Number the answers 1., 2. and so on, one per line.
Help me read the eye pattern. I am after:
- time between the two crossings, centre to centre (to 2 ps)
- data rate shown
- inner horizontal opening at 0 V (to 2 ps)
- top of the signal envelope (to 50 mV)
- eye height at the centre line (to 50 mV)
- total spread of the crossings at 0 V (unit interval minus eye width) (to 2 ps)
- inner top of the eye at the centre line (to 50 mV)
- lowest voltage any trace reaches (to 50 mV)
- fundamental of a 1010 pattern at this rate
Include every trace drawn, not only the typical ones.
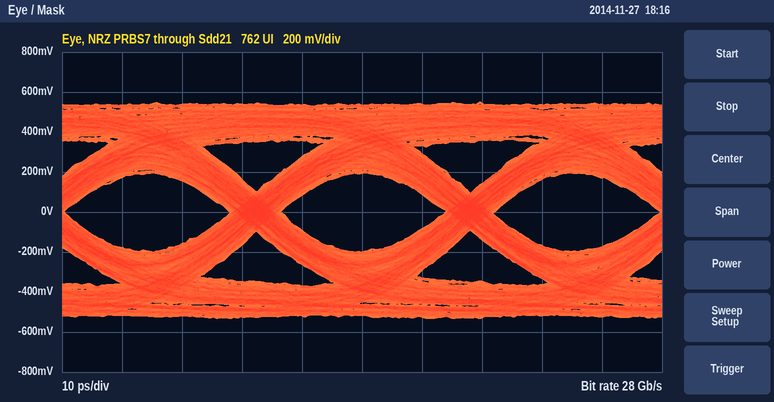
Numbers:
1. 36 ps
2. 28 Gb/s
3. 28 ps
4. 550 mV
5. 400 mV
6. 8 ps
7. 200 mV
8. -550 mV
9. 14 GHz
